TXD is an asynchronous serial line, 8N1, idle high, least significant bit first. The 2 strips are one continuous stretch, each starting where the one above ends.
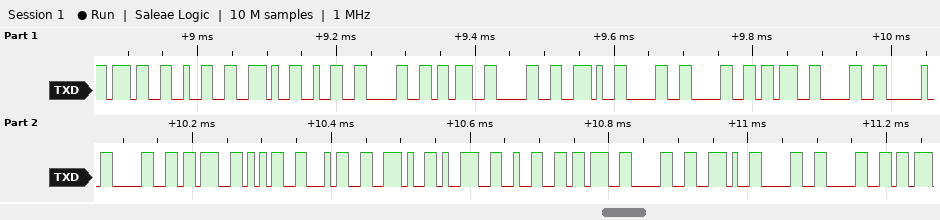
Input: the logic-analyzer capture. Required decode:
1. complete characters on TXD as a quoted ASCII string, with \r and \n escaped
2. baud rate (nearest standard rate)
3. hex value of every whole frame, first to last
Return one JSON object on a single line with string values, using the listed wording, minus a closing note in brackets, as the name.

{"complete characters on TXD as a quoted ASCII string, with \\r and \\n escaped": "\"72.20;0.00;0 0;54.92;0.00\"", "baud rate": "115200 baud", "hex value of every whole frame, first to last": "37 32 2E 32 30 3B 30 2E 30 30 3B 30 20 30 3B 35 34 2E 39 32 3B 30 2E 30 30"}
